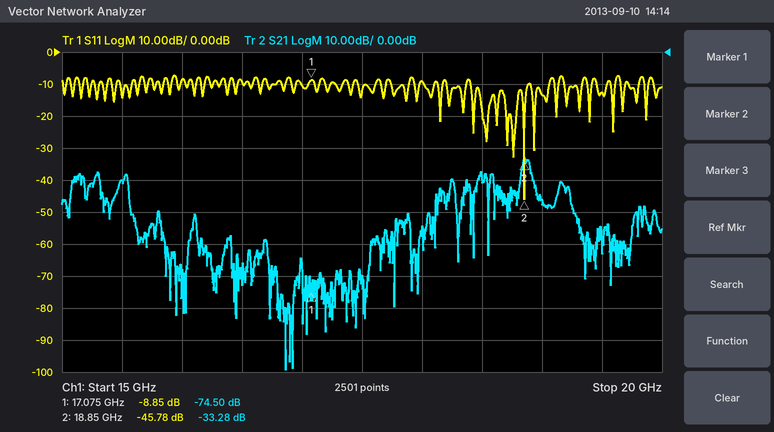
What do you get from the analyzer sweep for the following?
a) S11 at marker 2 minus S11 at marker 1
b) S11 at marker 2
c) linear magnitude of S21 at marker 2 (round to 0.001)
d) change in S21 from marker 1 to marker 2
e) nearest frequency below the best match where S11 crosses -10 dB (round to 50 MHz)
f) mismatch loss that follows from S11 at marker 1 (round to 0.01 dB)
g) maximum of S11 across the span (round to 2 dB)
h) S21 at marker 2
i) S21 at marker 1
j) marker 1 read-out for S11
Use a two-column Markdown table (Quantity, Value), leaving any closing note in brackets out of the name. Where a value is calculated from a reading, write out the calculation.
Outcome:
| Quantity | Value |
|---|---|
| S11 at marker 2 minus S11 at marker 1 | -45.78 − (-8.85) = -36.93 dB |
| S11 at marker 2 | -45.78 dB |
| linear magnitude of S21 at marker 2 | 10^(-33.28/20) ≈ 0.022 |
| change in S21 from marker 1 to marker 2 | -33.28 − (-74.5) = 41.22 dB |
| nearest frequency below the best match where S11 crosses -10 dB | 18.40 GHz |
| mismatch loss that follows from S11 at marker 1 | −10 log10(1 − 10^(-8.85/10)) ≈ 0.61 dB |
| maximum of S11 across the span | -8 dB |
| S21 at marker 2 | -33.28 dB |
| S21 at marker 1 | -74.50 dB |
| marker 1 read-out for S11 | -8.85 dB |
